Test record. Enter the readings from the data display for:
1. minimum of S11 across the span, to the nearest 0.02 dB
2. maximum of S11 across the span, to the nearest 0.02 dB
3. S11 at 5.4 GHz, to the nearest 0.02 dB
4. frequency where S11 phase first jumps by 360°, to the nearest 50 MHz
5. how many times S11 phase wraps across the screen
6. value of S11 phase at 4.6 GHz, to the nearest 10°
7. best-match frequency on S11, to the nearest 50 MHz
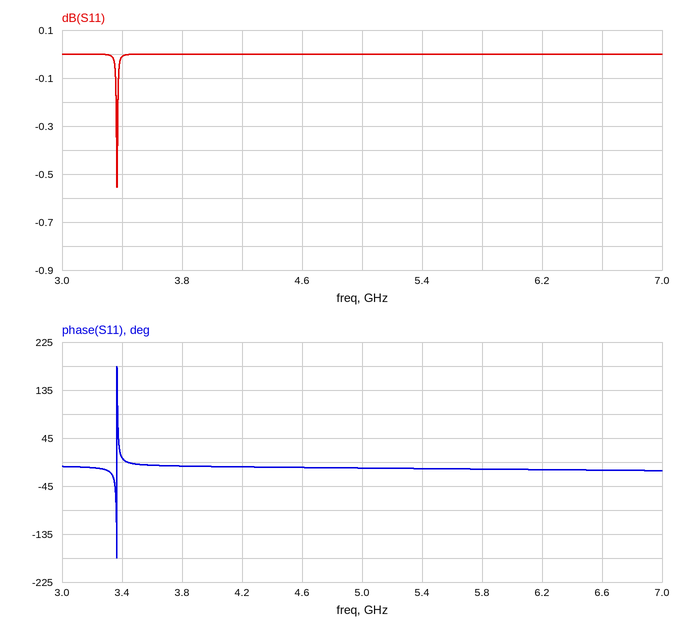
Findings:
-0.56 dB
0.00 dB
0.00 dB
3.35 GHz
1
-10°
3.35 GHz
